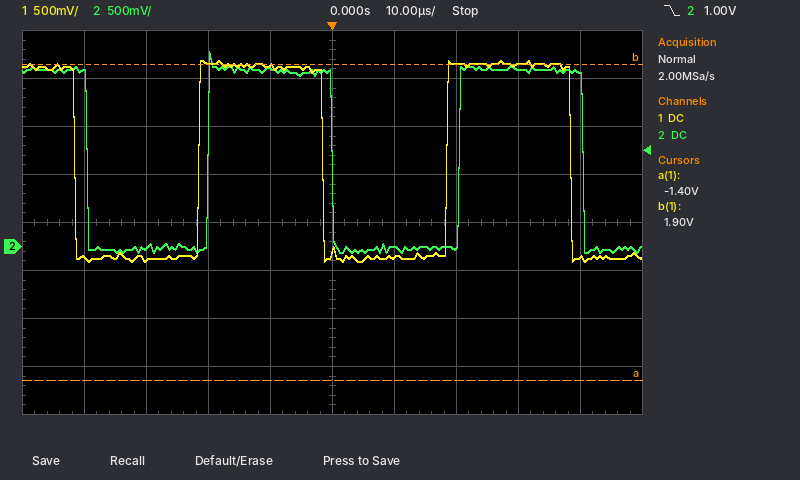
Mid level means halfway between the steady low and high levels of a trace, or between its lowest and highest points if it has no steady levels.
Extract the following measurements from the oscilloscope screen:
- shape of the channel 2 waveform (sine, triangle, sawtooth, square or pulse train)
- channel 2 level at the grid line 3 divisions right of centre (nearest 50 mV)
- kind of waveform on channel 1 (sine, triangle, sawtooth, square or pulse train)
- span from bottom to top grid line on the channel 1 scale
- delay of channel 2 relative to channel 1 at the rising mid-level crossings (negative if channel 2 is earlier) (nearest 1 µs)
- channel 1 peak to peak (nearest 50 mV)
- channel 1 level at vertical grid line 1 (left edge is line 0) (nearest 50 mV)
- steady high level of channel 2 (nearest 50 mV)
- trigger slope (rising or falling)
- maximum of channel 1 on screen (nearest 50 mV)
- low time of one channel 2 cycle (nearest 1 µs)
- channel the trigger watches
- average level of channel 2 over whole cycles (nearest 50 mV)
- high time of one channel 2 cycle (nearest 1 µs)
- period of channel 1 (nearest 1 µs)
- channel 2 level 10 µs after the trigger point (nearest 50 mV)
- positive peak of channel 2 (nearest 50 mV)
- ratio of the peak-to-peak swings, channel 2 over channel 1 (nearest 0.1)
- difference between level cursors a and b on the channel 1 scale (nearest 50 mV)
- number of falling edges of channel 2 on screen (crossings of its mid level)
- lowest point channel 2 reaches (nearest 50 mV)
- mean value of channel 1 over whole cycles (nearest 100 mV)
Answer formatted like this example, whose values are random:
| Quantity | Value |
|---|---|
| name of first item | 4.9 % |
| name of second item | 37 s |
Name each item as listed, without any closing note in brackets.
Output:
| Quantity | Value |
|---|---|
| shape of the channel 2 waveform | square |
| channel 2 level at the grid line 3 divisions right of centre | 1.85 V |
| kind of waveform on channel 1 | square |
| span from bottom to top grid line on the channel 1 scale | 4 V |
| delay of channel 2 relative to channel 1 at the rising mid-level crossings (negative if channel 2 is earlier) | +2 µs |
| channel 1 peak to peak | 2.10 V |
| channel 1 level at vertical grid line 1 (left edge is line 0) | -100 mV |
| steady high level of channel 2 | 1.85 V |
| trigger slope | falling |
| maximum of channel 1 on screen | 1.95 V |
| low time of one channel 2 cycle | 20 µs |
| channel the trigger watches | channel 2 |
| average level of channel 2 over whole cycles | 900 mV |
| high time of one channel 2 cycle | 20 µs |
| period of channel 1 | 40 µs |
| channel 2 level 10 µs after the trigger point | 0 mV |
| positive peak of channel 2 | 2.05 V |
| ratio of the peak-to-peak swings, channel 2 over channel 1 | 1.0 |
| difference between level cursors a and b on the channel 1 scale | 3.30 V |
| number of falling edges of channel 2 on screen | 3 |
| lowest point channel 2 reaches | -50 mV |
| mean value of channel 1 over whole cycles | 900 mV |
